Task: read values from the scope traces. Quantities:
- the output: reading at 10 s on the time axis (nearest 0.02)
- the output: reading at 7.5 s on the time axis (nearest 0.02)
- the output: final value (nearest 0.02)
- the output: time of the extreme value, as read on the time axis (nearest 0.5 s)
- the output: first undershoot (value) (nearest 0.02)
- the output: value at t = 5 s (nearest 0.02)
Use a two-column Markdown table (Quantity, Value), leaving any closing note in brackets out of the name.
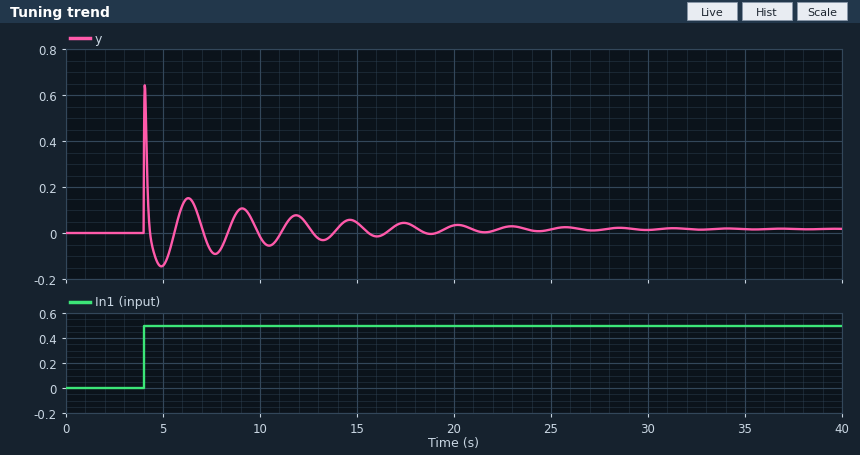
| Quantity | Value |
|---|---|
| the output: reading at 10 s on the time axis | -0.02 |
| the output: reading at 7.5 s on the time axis | -0.08 |
| the output: final value | 0.02 |
| the output: time of the extreme value, as read on the time axis | 4.0 s |
| the output: first undershoot (value) | -0.14 |
| the output: value at t = 5 s | -0.14 |
